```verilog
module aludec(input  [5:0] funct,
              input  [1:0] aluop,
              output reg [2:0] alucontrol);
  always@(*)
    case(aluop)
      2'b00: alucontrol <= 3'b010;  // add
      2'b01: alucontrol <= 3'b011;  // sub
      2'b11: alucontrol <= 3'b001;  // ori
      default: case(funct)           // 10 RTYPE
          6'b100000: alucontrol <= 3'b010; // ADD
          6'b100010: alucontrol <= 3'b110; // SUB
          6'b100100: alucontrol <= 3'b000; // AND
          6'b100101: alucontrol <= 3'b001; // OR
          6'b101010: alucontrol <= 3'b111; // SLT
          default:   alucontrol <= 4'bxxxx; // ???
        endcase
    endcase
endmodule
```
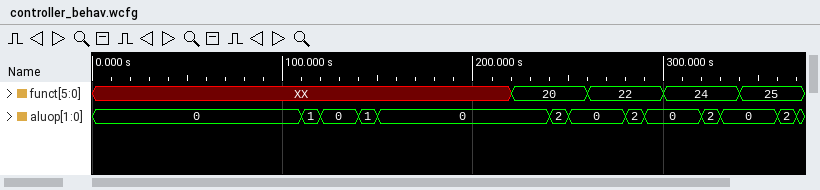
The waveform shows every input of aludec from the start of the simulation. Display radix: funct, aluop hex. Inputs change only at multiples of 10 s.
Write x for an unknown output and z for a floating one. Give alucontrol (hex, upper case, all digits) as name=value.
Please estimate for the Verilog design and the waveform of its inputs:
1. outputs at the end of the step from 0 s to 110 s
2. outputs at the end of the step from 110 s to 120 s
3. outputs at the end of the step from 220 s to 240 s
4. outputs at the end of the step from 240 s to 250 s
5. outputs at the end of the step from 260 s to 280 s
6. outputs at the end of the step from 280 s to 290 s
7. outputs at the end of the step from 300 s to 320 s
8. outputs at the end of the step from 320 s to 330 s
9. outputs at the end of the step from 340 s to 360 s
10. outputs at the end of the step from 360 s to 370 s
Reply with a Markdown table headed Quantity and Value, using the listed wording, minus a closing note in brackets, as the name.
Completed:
| Quantity | Value |
|---|---|
| outputs at the end of the step from 0 s to 110 s | alucontrol=2 |
| outputs at the end of the step from 110 s to 120 s | alucontrol=3 |
| outputs at the end of the step from 220 s to 240 s | alucontrol=2 |
| outputs at the end of the step from 240 s to 250 s | alucontrol=2 |
| outputs at the end of the step from 260 s to 280 s | alucontrol=2 |
| outputs at the end of the step from 280 s to 290 s | alucontrol=6 |
| outputs at the end of the step from 300 s to 320 s | alucontrol=2 |
| outputs at the end of the step from 320 s to 330 s | alucontrol=0 |
| outputs at the end of the step from 340 s to 360 s | alucontrol=2 |
| outputs at the end of the step from 360 s to 370 s | alucontrol=1 |
